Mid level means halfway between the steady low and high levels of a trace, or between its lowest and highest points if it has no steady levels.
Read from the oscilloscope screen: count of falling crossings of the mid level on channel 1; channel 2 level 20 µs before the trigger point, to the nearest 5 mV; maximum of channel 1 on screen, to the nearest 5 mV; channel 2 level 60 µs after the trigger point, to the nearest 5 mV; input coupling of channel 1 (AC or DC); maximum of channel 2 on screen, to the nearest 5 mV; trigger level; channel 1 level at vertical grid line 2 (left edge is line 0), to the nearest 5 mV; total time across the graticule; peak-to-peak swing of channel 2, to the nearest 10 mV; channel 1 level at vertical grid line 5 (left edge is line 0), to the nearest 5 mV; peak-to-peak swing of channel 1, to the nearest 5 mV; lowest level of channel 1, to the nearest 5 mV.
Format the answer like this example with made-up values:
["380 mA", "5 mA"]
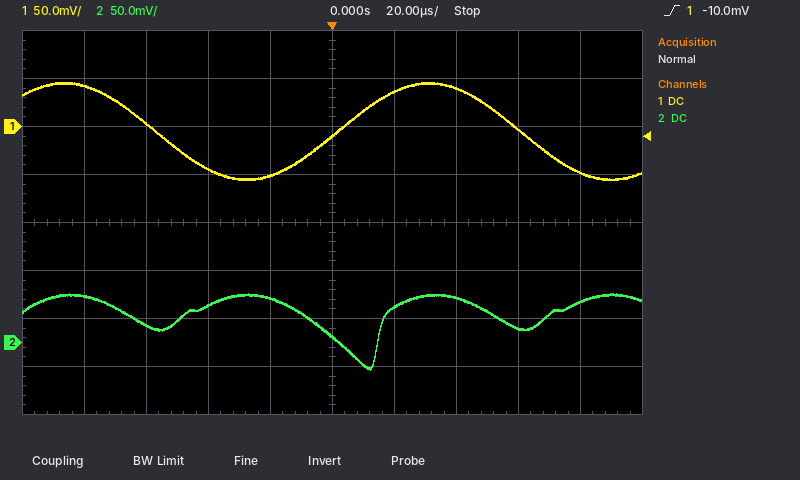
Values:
["2", "45 mV", "45 mV", "15 mV", "DC", "50 mV", "-10.0 mV", "5 mV", "200 µs", "80 mV", "-10 mV", "100 mV", "-55 mV"]
